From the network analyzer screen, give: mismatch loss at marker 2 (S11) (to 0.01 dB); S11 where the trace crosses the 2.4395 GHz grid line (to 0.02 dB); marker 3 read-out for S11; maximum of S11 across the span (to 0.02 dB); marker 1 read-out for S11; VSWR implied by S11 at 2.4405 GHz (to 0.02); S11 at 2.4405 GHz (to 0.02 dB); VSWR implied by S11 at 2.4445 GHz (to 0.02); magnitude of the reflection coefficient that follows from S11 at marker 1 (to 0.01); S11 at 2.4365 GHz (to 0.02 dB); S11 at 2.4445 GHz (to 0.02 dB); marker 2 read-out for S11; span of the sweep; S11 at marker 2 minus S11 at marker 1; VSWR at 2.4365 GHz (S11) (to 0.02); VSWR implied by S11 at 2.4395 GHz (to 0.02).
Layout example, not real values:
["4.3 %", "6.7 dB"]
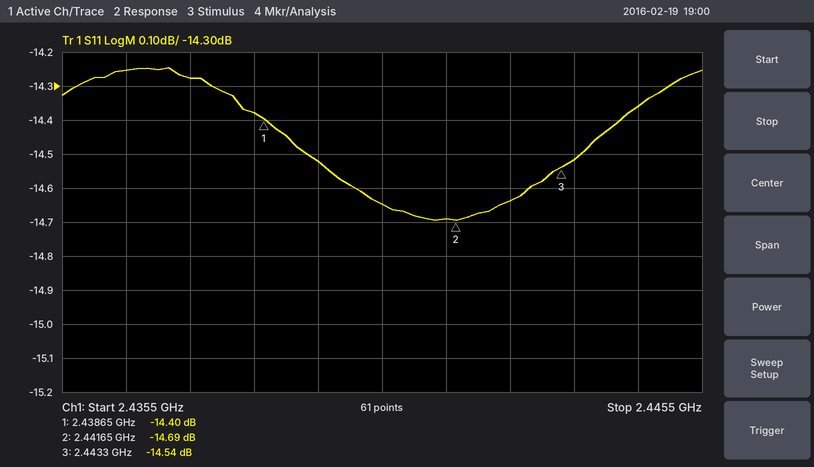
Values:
["0.15 dB", "-14.52 dB", "-14.54 dB", "-14.24 dB", "-14.40 dB", "1.46", "-14.64 dB", "1.48", "0.19", "-14.26 dB", "-14.36 dB", "-14.69 dB", "10 MHz", "-0.29 dB", "1.48", "1.46"]
